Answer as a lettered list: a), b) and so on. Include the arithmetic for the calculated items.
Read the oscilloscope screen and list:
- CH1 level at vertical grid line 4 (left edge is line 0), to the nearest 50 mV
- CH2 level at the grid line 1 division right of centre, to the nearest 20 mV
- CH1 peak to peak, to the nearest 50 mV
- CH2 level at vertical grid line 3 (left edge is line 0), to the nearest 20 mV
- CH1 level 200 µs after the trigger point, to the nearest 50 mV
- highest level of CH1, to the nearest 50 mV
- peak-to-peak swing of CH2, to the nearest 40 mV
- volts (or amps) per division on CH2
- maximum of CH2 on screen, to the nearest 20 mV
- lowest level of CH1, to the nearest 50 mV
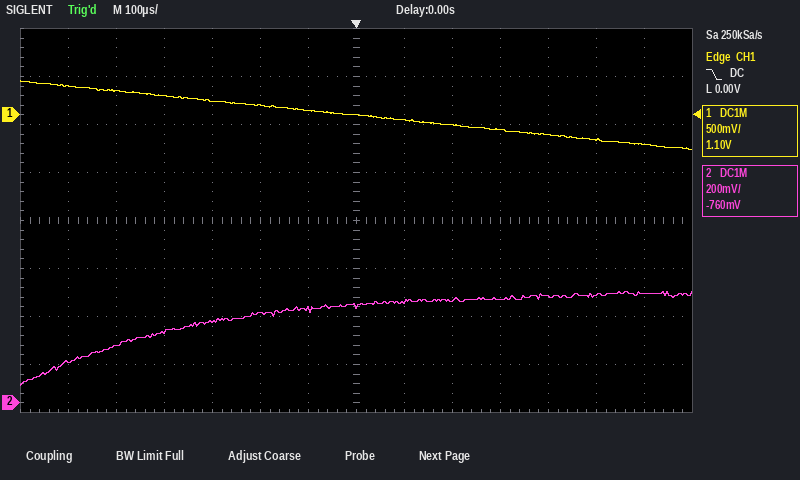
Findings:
a) 150 mV
b) 420 mV
c) 350 mV − (-350 mV) = 700 mV
d) 300 mV
e) -100 mV
f) 350 mV
g) 400 mV
h) 200 mV
i) 460 mV
j) -350 mV
